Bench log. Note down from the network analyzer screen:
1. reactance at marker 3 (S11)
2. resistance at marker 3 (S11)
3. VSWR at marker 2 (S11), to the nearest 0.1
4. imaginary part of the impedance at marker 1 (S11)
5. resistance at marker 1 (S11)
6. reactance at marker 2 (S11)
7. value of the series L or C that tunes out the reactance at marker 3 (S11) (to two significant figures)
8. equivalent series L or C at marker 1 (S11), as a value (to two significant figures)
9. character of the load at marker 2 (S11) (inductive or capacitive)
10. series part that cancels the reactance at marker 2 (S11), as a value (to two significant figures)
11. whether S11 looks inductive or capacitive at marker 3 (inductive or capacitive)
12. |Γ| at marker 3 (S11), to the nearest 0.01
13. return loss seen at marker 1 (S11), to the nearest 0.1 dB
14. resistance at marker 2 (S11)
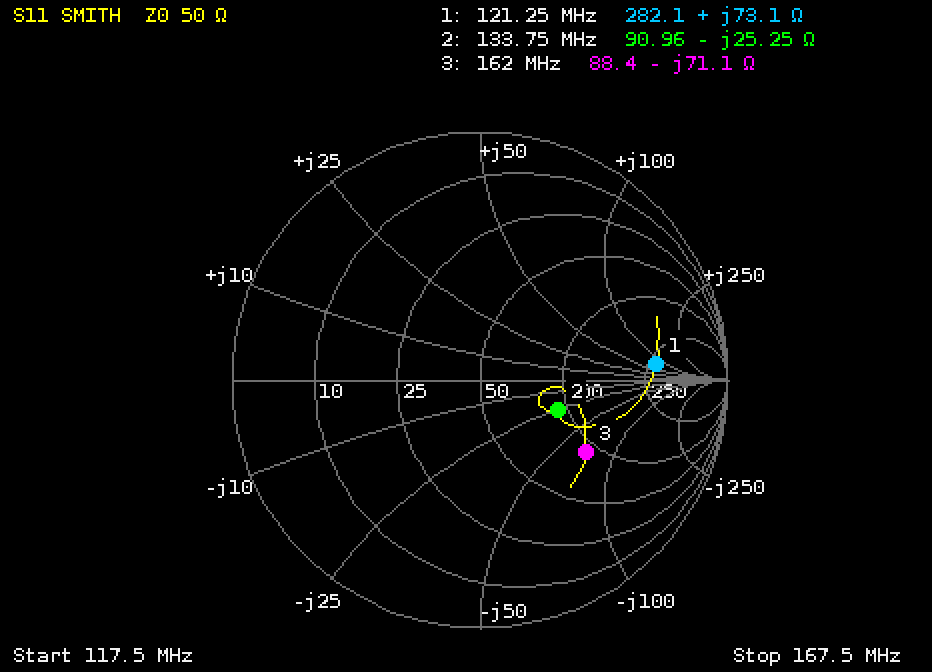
-71.1 Ω
88.4 Ω
2.0
+73.1 Ω
282.1 Ω
-25.25 Ω
70 nH
96 nH
capacitive
30 nH
capacitive
0.52
2.9 dB
90.96 Ω
